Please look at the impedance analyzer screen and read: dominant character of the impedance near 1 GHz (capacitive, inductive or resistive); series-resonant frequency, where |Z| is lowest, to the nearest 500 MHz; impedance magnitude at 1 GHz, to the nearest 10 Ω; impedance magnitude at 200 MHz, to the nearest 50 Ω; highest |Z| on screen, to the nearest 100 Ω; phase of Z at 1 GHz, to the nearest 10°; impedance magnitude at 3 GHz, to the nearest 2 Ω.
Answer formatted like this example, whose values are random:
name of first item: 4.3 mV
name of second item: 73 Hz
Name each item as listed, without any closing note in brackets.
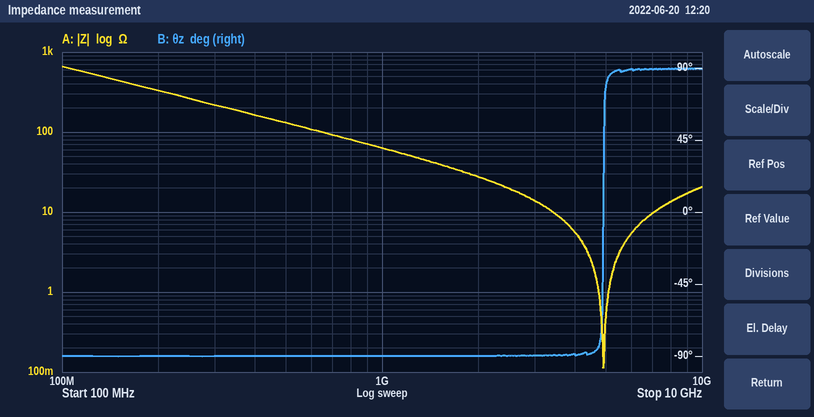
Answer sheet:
dominant character of the impedance near 1 GHz: capacitive
series-resonant frequency, where |Z| is lowest, to the nearest 500 MHz: 5.0 GHz
impedance magnitude at 1 GHz, to the nearest 10 Ω: 60 Ω
impedance magnitude at 200 MHz, to the nearest 50 Ω: 350 Ω
highest |Z| on screen, to the nearest 100 Ω: 700 Ω
phase of Z at 1 GHz, to the nearest 10°: -90°
impedance magnitude at 3 GHz, to the nearest 2 Ω: 14 Ω
